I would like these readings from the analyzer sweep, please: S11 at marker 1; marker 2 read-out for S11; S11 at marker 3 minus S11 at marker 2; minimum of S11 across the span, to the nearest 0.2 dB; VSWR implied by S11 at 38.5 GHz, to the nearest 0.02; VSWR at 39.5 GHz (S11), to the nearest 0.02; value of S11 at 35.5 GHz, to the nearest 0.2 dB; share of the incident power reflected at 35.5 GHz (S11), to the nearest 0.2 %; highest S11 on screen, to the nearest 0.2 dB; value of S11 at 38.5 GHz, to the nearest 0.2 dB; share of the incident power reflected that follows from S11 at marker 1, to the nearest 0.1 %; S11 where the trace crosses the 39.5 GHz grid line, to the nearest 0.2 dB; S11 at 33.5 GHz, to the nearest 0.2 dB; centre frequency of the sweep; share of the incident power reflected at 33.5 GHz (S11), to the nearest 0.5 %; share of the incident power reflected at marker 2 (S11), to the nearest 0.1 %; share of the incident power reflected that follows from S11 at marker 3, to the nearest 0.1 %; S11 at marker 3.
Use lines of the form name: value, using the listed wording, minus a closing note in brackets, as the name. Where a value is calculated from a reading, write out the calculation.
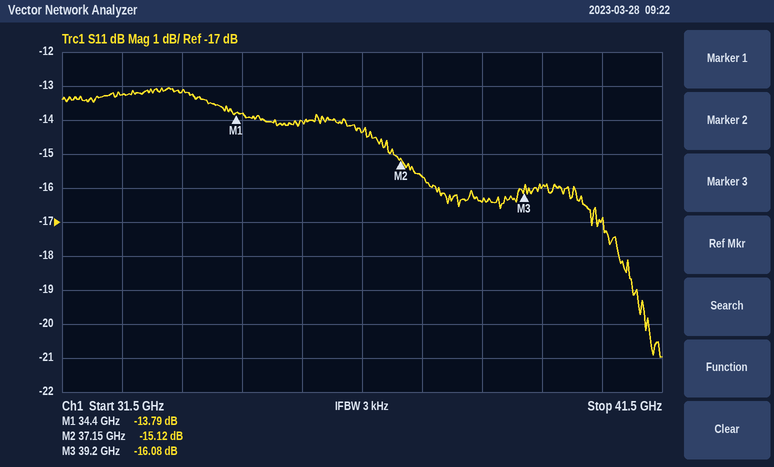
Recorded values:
S11 at marker 1: -13.79 dB
marker 2 read-out for S11: -15.12 dB
S11 at marker 3 minus S11 at marker 2: -16.08 − (-15.12) = -0.96 dB
minimum of S11 across the span, to the nearest 0.2 dB: -21.0 dB
VSWR implied by S11 at 38.5 GHz, to the nearest 0.02: |Γ| = 10^(-16.4/20) = 0.1514; VSWR = (1 + 0.1514)/(1 − 0.1514) ≈ 1.36
VSWR at 39.5 GHz (S11), to the nearest 0.02: |Γ| = 10^(-16/20) = 0.1585; VSWR = (1 + 0.1585)/(1 − 0.1585) ≈ 1.38
value of S11 at 35.5 GHz, to the nearest 0.2 dB: -14.0 dB
share of the incident power reflected at 35.5 GHz (S11), to the nearest 0.2 %: 10^(-14/10) ≈ 4.0 %
highest S11 on screen, to the nearest 0.2 dB: -13.0 dB
value of S11 at 38.5 GHz, to the nearest 0.2 dB: -16.4 dB
share of the incident power reflected that follows from S11 at marker 1, to the nearest 0.1 %: 10^(-13.79/10) ≈ 4.2 %
S11 where the trace crosses the 39.5 GHz grid line, to the nearest 0.2 dB: -16.0 dB
S11 at 33.5 GHz, to the nearest 0.2 dB: -13.2 dB
centre frequency of the sweep: 36.5 GHz
share of the incident power reflected at 33.5 GHz (S11), to the nearest 0.5 %: 10^(-13.2/10) ≈ 4.79 %, so 5.0 % to the nearest 0.5 %
share of the incident power reflected at marker 2 (S11), to the nearest 0.1 %: 10^(-15.12/10) ≈ 3.1 %
share of the incident power reflected that follows from S11 at marker 3, to the nearest 0.1 %: 10^(-16.08/10) ≈ 2.5 %
S11 at marker 3: -16.08 dB
